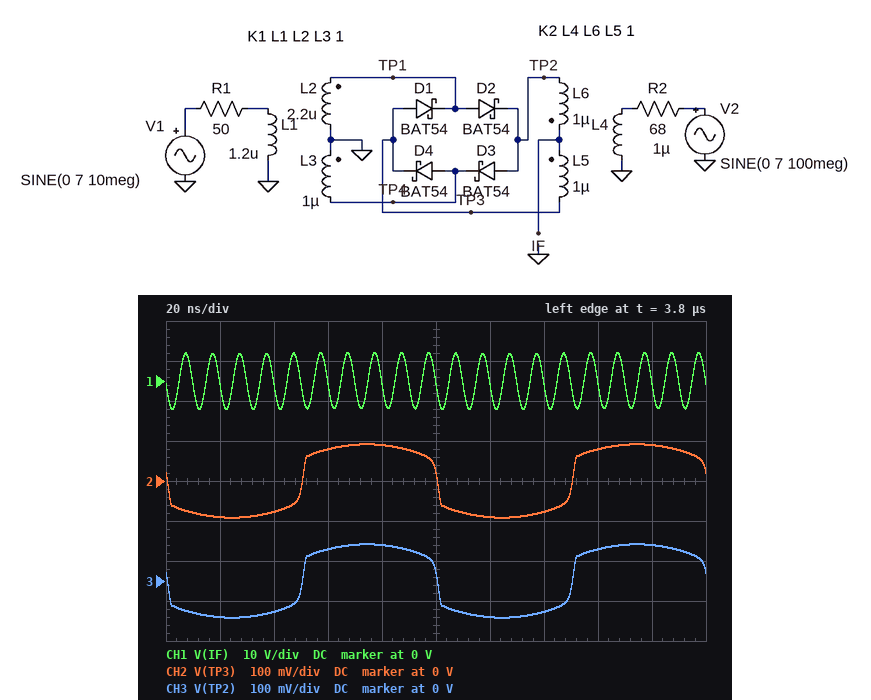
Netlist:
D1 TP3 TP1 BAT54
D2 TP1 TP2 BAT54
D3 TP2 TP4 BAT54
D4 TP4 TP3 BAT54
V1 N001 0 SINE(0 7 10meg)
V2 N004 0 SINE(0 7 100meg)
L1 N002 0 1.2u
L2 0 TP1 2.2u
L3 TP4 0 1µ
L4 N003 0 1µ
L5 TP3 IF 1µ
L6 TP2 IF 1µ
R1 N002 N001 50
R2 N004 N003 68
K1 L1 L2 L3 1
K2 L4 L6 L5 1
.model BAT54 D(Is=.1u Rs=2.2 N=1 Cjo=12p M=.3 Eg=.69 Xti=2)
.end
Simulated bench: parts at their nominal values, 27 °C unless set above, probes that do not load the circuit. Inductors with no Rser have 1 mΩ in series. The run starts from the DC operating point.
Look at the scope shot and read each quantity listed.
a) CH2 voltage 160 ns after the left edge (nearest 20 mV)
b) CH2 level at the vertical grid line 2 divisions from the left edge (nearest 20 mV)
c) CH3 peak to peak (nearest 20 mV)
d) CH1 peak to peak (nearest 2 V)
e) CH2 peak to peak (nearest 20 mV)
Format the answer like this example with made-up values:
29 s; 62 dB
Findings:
80 mV; -80 mV; 180 mV; 14 V; 180 mV
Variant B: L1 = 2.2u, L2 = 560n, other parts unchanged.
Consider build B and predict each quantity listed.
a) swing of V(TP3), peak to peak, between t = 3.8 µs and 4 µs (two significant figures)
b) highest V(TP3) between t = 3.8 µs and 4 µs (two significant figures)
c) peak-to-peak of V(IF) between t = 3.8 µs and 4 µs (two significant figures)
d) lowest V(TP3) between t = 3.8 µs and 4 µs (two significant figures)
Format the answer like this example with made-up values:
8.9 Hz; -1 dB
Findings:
170 mV; 84 mV; 14 V; -84 mV
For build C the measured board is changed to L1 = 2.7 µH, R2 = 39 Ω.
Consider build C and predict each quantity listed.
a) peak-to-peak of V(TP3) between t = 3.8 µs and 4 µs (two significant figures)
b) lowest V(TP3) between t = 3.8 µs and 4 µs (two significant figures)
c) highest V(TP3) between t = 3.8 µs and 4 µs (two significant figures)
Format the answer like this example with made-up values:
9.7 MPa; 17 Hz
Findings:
210 mV; -100 mV; 100 mV
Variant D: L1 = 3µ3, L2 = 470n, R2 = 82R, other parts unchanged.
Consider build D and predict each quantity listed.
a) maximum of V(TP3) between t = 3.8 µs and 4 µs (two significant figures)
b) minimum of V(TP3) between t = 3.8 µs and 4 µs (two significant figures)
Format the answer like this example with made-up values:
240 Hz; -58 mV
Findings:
120 mV; -120 mV
